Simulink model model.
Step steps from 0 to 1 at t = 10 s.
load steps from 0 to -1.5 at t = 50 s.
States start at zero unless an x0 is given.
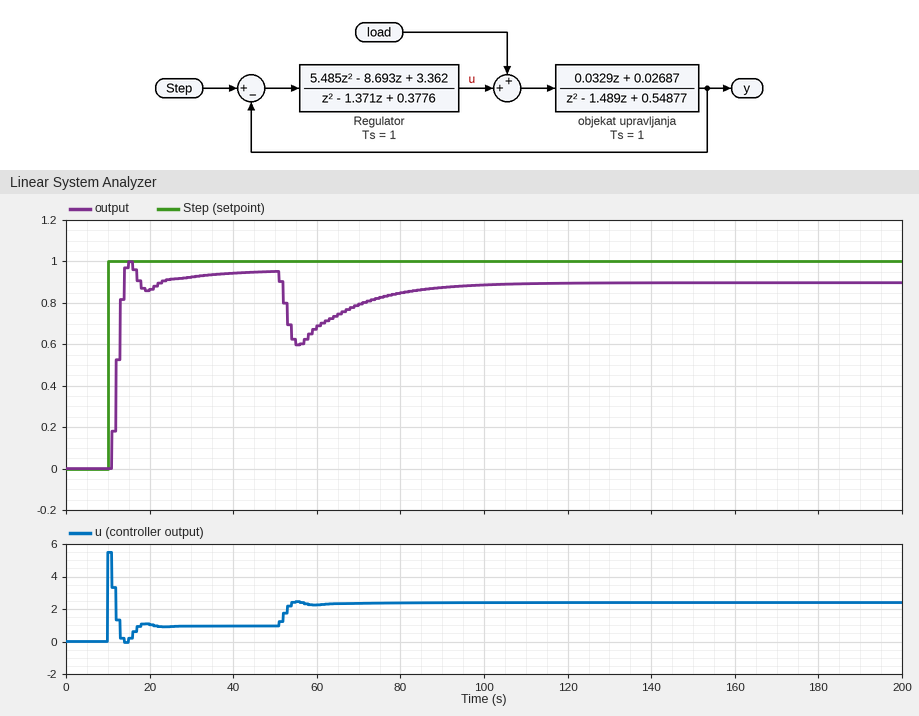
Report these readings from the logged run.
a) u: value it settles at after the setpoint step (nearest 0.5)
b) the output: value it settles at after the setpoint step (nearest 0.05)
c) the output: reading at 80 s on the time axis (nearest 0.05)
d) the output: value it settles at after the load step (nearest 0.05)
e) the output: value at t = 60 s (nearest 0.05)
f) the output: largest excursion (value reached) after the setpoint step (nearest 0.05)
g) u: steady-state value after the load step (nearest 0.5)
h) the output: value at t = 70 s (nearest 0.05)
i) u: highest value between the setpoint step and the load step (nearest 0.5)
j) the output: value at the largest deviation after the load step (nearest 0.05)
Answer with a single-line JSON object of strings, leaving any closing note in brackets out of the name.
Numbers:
{"u: value it settles at after the setpoint step": "1.0", "the output: value it settles at after the setpoint step": "0.95", "the output: reading at 80 s on the time axis": "0.85", "the output: value it settles at after the load step": "0.90", "the output: value at t = 60 s": "0.70", "the output: largest excursion (value reached) after the setpoint step": "1.00", "u: steady-state value after the load step": "2.5", "the output: value at t = 70 s": "0.80", "u: highest value between the setpoint step and the load step": "5.5", "the output: value at the largest deviation after the load step": "0.60"}
